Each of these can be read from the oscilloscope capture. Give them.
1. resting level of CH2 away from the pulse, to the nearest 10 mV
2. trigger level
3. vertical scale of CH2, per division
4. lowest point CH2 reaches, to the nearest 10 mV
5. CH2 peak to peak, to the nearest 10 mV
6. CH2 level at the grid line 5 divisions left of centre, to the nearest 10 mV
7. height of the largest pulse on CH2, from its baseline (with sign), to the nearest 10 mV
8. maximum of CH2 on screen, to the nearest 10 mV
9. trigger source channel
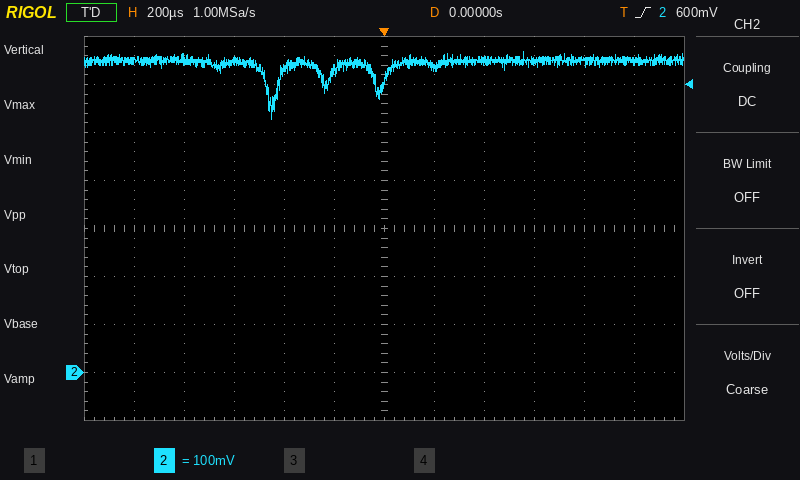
650 mV
600 mV
100 mV
530 mV
140 mV
650 mV
-120 mV
670 mV
CH2
